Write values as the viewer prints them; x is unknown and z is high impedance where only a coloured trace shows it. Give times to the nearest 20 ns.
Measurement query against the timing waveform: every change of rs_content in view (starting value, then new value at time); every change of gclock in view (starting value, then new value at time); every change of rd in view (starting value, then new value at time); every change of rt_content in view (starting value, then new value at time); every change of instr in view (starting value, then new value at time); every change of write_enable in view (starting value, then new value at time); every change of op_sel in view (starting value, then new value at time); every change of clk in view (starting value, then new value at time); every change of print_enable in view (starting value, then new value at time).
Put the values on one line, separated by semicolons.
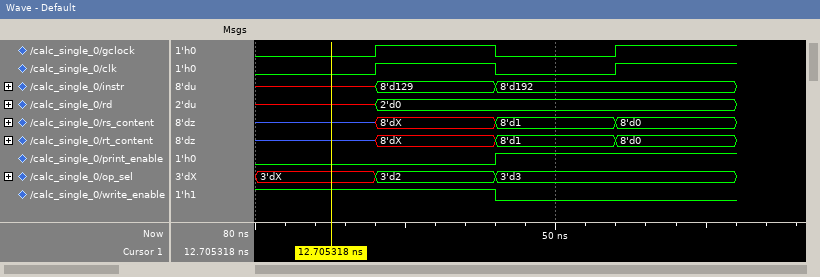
z, 8'dX at 20 ns, 8'd1 at 40 ns, 8'd0 at 60 ns; 0, 1 at 20 ns, 0 at 40 ns, 1 at 60 ns; x, 2'd0 at 20 ns; z, 8'dX at 20 ns, 8'd1 at 40 ns, 8'd0 at 60 ns; x, 8'd129 at 20 ns, 8'd192 at 40 ns; 1, 0 at 40 ns; 3'dX, 3'd2 at 20 ns, 3'd3 at 40 ns; 0, 1 at 20 ns, 0 at 40 ns, 1 at 60 ns; 0, 1 at 40 ns
